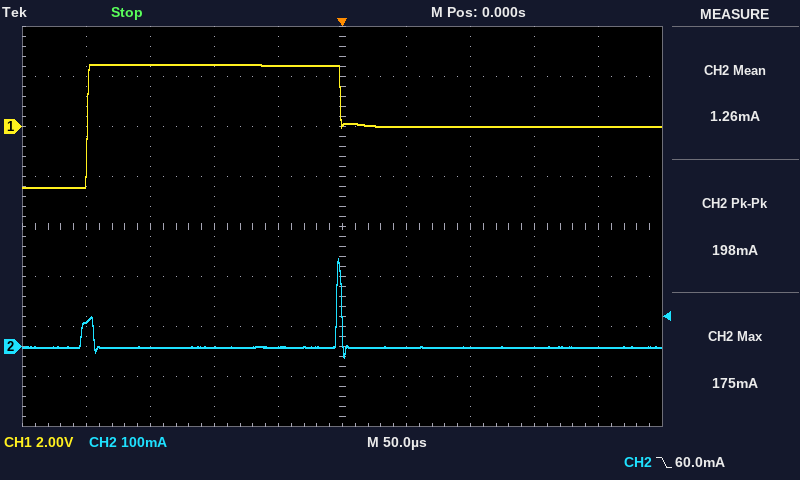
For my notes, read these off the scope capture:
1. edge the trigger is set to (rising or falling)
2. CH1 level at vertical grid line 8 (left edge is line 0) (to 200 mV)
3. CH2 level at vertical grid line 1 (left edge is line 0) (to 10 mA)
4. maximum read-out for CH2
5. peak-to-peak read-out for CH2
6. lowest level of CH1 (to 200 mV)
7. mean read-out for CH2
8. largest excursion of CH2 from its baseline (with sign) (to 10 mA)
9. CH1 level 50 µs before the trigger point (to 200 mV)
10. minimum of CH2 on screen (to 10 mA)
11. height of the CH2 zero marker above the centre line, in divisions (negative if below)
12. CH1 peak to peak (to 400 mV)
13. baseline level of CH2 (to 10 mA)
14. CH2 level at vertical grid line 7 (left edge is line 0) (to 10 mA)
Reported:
falling
0.0 V
50 mA
175 mA
198 mA
-2.4 V
1.26 mA
+180 mA
2.4 V
-20 mA
-2.4 div
4.8 V
0 mA
0 mA
